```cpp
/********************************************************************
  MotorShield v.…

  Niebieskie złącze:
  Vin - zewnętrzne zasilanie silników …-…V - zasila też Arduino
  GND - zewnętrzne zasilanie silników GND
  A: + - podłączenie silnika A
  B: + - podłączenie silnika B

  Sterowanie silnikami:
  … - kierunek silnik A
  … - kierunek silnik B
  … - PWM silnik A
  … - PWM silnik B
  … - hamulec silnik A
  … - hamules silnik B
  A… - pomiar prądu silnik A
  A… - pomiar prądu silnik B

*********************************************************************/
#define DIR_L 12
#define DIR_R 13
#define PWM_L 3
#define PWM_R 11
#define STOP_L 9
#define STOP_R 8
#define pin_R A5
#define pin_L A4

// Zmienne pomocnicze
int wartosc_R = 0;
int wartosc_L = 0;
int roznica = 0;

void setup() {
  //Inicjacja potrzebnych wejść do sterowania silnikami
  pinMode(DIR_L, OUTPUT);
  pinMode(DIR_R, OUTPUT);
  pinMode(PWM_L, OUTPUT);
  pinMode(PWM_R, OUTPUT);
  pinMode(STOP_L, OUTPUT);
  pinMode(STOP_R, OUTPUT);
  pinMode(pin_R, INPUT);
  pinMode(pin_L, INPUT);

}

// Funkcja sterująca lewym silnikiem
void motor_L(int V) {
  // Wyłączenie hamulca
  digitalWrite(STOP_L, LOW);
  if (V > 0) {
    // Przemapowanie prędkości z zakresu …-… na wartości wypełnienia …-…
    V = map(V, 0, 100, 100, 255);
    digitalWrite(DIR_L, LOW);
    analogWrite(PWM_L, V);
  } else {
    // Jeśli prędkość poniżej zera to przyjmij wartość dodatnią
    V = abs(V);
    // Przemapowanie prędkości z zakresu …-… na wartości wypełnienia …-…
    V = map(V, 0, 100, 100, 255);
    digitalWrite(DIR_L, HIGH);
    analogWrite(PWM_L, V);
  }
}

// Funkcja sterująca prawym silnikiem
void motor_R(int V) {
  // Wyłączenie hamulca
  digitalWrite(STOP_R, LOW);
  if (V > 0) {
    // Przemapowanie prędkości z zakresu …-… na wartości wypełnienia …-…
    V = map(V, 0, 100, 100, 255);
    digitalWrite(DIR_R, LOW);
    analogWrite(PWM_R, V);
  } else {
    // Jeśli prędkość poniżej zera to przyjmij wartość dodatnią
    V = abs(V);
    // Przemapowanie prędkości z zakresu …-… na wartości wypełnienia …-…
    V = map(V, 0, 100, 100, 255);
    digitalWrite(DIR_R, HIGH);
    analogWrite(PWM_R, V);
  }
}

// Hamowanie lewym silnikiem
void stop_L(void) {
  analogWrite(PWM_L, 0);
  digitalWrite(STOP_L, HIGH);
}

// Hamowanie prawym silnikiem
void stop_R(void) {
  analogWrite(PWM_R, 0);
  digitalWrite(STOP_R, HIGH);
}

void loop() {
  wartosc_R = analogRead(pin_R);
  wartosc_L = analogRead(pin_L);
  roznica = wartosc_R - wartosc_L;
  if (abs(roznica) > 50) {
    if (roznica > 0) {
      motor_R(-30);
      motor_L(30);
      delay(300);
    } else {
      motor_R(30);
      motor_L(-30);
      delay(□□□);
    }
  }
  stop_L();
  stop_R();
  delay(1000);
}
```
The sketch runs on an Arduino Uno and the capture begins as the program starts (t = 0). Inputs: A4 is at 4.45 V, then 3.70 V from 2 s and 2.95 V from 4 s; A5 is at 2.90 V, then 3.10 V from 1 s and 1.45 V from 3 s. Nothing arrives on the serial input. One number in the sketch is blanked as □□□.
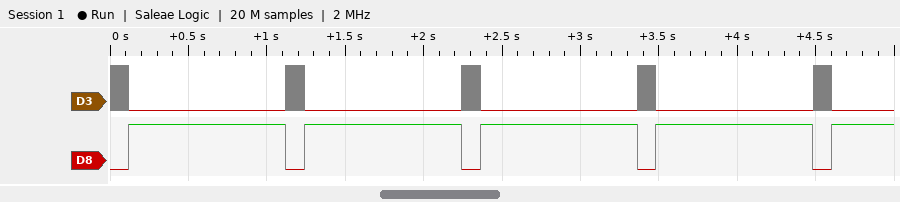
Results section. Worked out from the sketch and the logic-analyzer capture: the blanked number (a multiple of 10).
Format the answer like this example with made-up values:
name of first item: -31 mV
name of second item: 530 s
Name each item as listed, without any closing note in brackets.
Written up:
the blanked number: 120
